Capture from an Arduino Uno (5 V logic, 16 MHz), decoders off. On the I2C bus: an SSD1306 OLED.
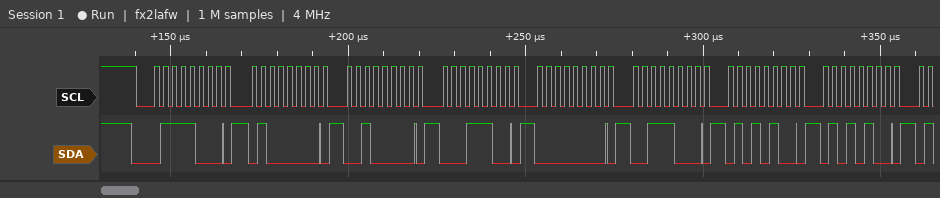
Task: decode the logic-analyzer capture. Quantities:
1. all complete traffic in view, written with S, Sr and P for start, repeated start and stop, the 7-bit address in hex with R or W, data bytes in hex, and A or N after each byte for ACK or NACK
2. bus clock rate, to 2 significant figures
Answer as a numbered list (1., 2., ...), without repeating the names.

1. S 3CW A 40 A 20 A 1C A 00 A 38 A 54 A 54 A
2. 400 kHz
